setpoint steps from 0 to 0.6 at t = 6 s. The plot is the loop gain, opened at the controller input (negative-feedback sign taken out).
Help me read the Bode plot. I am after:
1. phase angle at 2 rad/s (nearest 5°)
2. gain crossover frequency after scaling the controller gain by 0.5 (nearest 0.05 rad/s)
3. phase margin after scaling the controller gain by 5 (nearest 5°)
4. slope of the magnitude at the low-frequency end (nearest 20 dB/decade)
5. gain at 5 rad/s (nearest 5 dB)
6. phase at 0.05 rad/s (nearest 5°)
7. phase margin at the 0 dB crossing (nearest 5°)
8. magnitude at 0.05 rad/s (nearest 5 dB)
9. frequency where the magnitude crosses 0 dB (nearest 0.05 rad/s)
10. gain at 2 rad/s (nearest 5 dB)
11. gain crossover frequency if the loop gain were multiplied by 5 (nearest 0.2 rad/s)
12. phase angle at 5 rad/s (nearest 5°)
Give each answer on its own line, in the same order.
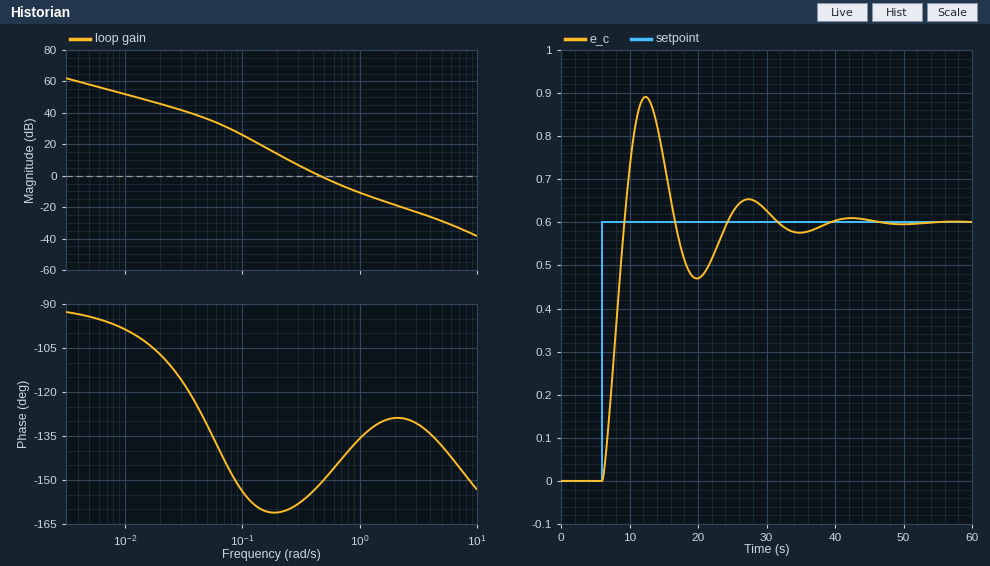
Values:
-130°
0.30 rad/s
50°
-20 dB/decade
-30 dB
-130°
30°
35 dB
0.45 rad/s
-20 dB
1.4 rad/s
-140°
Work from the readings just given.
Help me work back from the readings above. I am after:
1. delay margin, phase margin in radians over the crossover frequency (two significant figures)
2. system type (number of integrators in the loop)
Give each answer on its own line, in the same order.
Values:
1.2 s
1
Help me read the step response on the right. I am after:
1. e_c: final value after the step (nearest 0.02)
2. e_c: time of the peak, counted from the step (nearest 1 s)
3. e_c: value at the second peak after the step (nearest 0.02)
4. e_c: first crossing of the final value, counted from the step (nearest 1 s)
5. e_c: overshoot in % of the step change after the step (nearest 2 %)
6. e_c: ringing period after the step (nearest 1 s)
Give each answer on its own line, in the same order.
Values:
0.60
6 s
0.66
3 s
48 %
15 s
